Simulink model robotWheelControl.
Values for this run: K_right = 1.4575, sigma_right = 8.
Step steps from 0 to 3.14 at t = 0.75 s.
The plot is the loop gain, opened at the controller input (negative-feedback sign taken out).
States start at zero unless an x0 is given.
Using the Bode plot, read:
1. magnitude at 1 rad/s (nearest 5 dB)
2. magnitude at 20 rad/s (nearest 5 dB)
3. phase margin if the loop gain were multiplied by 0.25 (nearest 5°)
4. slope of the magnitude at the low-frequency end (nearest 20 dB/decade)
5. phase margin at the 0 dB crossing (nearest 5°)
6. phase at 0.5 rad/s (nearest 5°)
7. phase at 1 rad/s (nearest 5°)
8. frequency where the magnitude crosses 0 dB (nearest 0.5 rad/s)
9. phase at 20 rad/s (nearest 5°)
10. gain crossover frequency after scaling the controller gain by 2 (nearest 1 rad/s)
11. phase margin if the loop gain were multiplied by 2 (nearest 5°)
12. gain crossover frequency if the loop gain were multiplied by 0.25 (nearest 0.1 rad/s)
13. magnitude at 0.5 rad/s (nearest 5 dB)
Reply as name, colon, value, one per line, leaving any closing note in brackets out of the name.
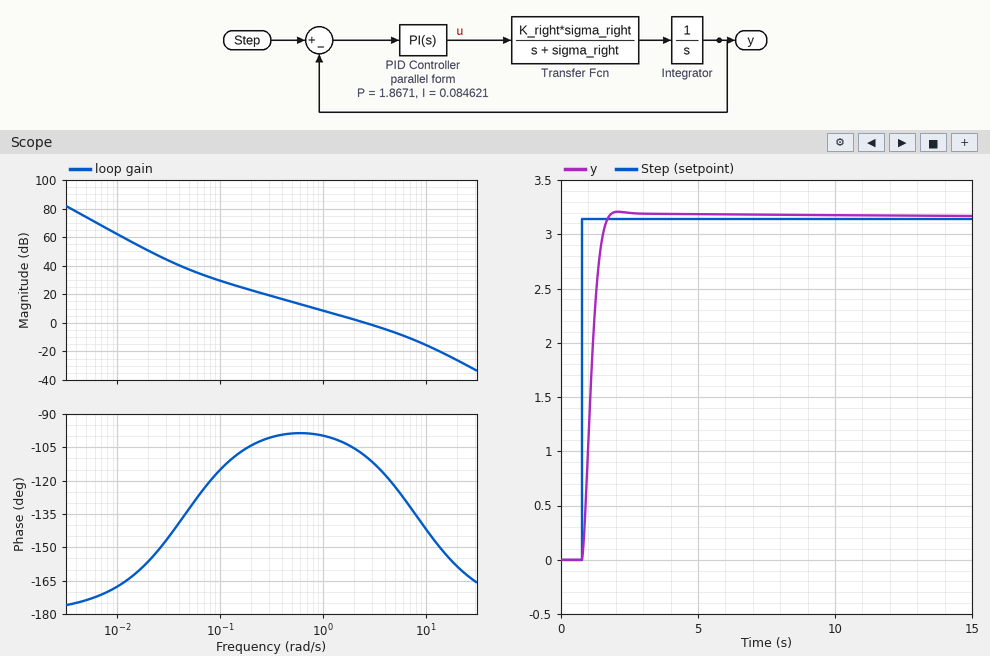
magnitude at 1 rad/s: 10 dB
magnitude at 20 rad/s: -25 dB
phase margin if the loop gain were multiplied by 0.25: 80°
slope of the magnitude at the low-frequency end: -40 dB/decade
phase margin at the 0 dB crossing: 70°
phase at 0.5 rad/s: -100°
phase at 1 rad/s: -100°
frequency where the magnitude crosses 0 dB: 2.5 rad/s
phase at 20 rad/s: -160°
gain crossover frequency after scaling the controller gain by 2: 5 rad/s
phase margin if the loop gain were multiplied by 2: 60°
gain crossover frequency if the loop gain were multiplied by 0.25: 0.7 rad/s
magnitude at 0.5 rad/s: 15 dB
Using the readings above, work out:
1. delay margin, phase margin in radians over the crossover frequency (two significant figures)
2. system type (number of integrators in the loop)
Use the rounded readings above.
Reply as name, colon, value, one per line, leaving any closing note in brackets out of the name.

delay margin, phase margin in radians over the crossover frequency: 0.49 s
system type: 2
